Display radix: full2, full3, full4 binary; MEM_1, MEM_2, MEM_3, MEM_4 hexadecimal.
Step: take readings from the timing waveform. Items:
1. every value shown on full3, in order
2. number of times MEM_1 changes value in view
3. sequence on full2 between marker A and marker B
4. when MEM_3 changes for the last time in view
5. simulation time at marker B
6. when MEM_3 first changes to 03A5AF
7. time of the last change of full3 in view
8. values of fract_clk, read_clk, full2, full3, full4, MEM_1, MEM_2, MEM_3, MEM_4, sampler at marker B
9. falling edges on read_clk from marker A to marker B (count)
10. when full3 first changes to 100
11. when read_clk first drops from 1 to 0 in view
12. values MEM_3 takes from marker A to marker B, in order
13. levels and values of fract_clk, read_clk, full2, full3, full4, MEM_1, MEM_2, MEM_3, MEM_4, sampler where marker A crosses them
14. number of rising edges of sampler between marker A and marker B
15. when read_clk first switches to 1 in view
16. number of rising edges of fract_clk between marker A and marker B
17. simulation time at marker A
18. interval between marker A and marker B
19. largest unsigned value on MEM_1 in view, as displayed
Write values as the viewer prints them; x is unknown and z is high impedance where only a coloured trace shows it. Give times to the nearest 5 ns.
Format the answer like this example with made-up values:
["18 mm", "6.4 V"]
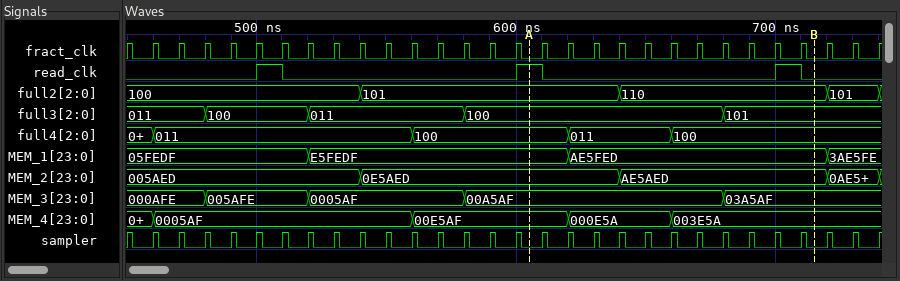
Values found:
["011, 100, 011, 100, 101", "3", "101, 110", "680 ns", "715 ns", "680 ns", "680 ns", "fract_clk=0, read_clk=0, full2=110, full3=101, full4=100, MEM_1=AE5FED, MEM_2=AE5AED, MEM_3=03A5AF, MEM_4=003E5A, sampler=0", "2", "480 ns", "510 ns", "00A5AF, 03A5AF", "fract_clk=0, read_clk=1, full2=101, full3=100, full4=100, MEM_1=E5FEDF, MEM_2=0E5AED, MEM_3=00A5AF, MEM_4=00E5AF, sampler=0", "11", "500 ns", "11", "605 ns", "110 ns", "E5FEDF"]
